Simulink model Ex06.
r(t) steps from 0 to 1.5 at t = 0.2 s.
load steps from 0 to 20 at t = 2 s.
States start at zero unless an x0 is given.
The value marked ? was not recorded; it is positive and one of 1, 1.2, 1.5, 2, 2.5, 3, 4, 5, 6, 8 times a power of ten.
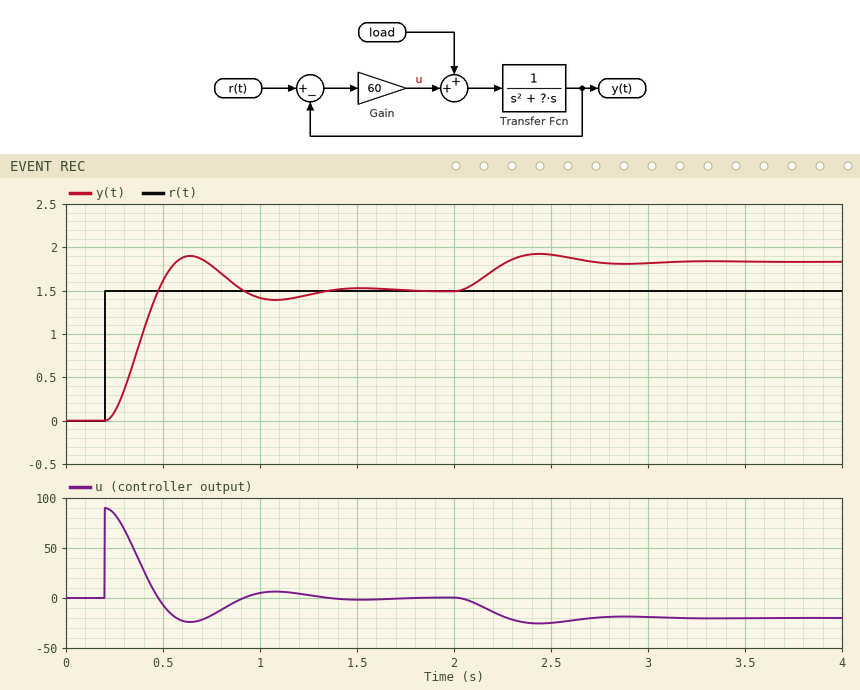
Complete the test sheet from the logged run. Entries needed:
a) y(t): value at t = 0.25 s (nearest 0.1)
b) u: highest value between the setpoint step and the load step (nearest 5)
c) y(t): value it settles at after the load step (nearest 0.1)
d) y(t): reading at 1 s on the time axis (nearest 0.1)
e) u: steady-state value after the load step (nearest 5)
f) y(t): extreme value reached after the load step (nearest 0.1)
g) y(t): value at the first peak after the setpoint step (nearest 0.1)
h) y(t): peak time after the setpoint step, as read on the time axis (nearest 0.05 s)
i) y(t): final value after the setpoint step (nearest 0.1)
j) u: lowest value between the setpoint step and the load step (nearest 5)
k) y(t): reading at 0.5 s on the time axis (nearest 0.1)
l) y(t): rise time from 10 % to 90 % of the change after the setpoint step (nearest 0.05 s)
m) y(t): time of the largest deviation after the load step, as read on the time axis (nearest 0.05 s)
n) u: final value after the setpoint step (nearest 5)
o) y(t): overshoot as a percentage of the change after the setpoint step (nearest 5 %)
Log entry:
0.1
90
1.8
1.4
-20
1.9
1.9
0.65 s
1.5
-25
1.6
0.20 s
2.45 s
0
25 %
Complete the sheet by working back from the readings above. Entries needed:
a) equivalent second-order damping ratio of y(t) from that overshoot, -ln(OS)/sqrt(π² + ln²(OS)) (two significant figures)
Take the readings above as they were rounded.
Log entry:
0.40
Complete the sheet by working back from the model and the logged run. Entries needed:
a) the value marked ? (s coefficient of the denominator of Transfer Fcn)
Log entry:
6
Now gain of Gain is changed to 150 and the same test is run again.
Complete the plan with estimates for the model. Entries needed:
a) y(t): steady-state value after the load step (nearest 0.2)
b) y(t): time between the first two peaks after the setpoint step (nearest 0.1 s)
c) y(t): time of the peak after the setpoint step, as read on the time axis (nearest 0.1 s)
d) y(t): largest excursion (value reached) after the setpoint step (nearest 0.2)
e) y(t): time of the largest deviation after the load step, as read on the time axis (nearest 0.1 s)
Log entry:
1.6
0.5 s
0.5 s
2.2
2.3 s
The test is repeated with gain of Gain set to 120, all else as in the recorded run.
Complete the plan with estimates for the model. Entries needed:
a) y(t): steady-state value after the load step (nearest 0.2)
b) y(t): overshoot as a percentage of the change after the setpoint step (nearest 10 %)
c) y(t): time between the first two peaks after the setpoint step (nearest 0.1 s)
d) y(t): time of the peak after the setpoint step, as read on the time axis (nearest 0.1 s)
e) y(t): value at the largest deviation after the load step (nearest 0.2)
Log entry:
1.6
40 %
0.6 s
0.5 s
1.8
